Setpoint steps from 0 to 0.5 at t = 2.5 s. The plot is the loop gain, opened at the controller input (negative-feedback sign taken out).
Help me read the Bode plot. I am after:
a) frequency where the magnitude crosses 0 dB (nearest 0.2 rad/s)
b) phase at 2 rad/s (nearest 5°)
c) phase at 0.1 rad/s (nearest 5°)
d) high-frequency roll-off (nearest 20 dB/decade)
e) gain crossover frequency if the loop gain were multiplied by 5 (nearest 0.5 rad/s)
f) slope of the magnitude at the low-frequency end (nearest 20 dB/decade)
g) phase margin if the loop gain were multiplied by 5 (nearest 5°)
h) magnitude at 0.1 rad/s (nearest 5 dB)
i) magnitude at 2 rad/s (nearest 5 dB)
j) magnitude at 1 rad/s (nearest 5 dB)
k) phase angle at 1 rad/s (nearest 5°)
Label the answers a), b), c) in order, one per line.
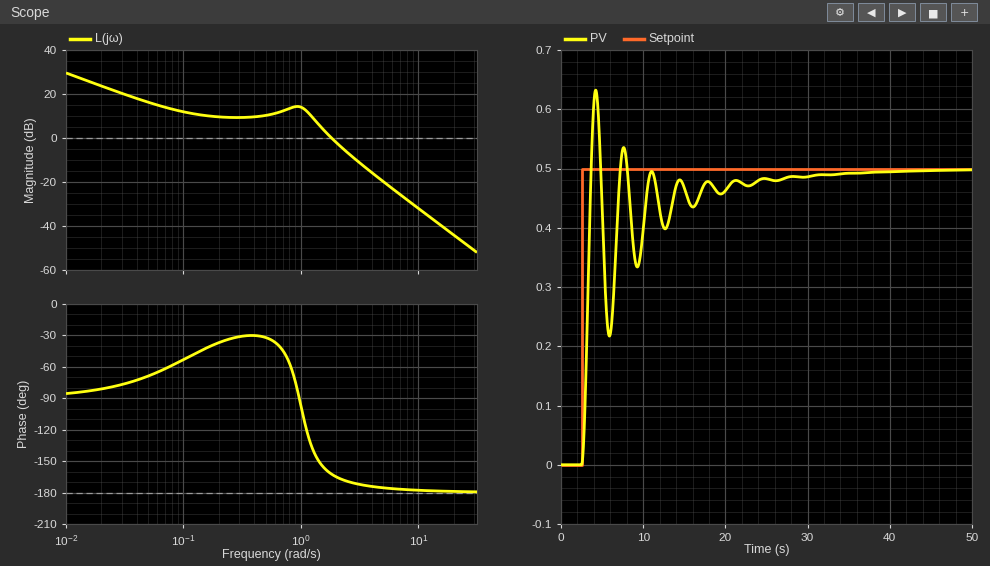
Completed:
a) 1.8 rad/s
b) -165°
c) -55°
d) -40 dB/decade
e) 3.5 rad/s
f) -20 dB/decade
g) 5°
h) 10 dB
i) 0 dB
j) 15 dB
k) -95°
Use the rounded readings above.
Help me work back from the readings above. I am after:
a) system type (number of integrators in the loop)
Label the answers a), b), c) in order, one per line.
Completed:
a) 1
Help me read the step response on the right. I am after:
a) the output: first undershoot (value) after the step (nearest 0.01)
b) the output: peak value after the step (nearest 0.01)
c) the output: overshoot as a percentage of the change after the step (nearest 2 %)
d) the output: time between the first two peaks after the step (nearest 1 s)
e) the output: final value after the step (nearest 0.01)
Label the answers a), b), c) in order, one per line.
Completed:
a) 0.22
b) 0.63
c) 26 %
d) 3 s
e) 0.50
